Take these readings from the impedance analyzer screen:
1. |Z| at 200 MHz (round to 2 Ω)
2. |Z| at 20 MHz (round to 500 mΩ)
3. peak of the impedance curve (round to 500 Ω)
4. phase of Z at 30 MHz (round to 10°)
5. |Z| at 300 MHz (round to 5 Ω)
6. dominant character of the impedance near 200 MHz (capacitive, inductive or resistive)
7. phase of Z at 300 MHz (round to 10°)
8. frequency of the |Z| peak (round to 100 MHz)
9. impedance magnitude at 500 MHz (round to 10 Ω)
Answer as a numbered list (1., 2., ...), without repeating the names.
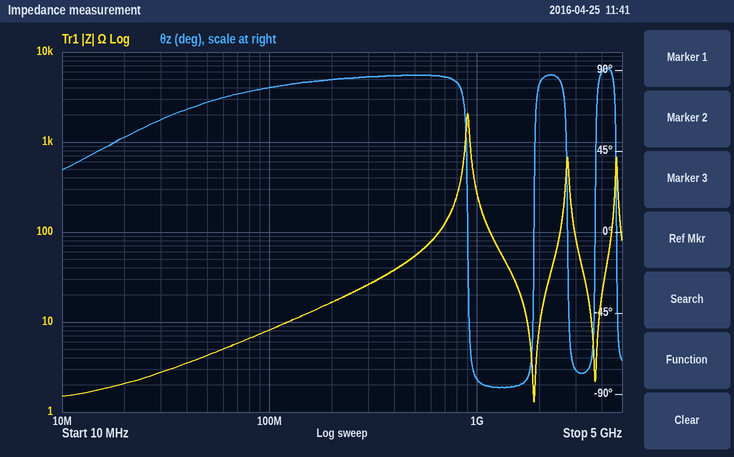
1. 16 Ω
2. 2.0 Ω
3. 2.0 kΩ
4. 60°
5. 25 Ω
6. inductive
7. 90°
8. 900 MHz
9. 50 Ω
